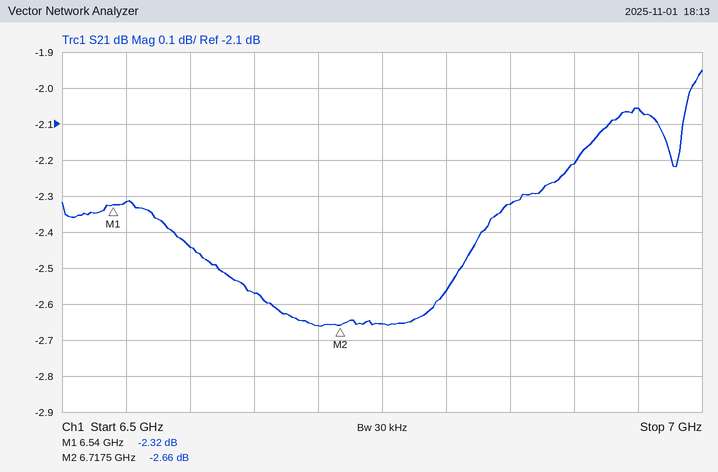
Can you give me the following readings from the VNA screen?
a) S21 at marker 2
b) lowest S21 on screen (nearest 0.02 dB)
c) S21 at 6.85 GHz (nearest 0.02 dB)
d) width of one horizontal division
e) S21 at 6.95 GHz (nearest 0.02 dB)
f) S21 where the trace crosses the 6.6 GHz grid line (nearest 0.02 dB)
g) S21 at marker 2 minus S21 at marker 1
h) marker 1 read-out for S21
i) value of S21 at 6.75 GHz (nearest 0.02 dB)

-2.66 dB
-2.66 dB
-2.32 dB
50 MHz
-2.06 dB
-2.44 dB
-0.34 dB
-2.32 dB
-2.66 dB
